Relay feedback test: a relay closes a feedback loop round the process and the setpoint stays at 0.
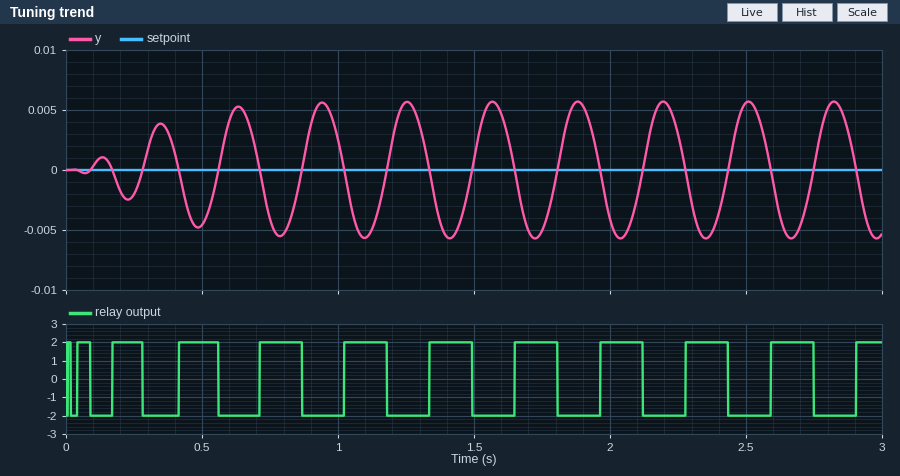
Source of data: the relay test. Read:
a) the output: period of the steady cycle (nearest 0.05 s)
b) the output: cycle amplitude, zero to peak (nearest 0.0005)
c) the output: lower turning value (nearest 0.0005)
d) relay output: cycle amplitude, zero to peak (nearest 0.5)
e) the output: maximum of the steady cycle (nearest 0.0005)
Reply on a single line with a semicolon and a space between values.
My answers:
0.30 s; 0.0055; -0.0055; 2.0; 0.0055
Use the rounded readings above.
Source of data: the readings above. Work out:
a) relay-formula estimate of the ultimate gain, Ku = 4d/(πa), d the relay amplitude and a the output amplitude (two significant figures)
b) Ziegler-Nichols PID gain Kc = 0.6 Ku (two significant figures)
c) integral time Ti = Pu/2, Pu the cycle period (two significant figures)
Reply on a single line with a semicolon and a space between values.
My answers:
460; 280; 0.15 s
